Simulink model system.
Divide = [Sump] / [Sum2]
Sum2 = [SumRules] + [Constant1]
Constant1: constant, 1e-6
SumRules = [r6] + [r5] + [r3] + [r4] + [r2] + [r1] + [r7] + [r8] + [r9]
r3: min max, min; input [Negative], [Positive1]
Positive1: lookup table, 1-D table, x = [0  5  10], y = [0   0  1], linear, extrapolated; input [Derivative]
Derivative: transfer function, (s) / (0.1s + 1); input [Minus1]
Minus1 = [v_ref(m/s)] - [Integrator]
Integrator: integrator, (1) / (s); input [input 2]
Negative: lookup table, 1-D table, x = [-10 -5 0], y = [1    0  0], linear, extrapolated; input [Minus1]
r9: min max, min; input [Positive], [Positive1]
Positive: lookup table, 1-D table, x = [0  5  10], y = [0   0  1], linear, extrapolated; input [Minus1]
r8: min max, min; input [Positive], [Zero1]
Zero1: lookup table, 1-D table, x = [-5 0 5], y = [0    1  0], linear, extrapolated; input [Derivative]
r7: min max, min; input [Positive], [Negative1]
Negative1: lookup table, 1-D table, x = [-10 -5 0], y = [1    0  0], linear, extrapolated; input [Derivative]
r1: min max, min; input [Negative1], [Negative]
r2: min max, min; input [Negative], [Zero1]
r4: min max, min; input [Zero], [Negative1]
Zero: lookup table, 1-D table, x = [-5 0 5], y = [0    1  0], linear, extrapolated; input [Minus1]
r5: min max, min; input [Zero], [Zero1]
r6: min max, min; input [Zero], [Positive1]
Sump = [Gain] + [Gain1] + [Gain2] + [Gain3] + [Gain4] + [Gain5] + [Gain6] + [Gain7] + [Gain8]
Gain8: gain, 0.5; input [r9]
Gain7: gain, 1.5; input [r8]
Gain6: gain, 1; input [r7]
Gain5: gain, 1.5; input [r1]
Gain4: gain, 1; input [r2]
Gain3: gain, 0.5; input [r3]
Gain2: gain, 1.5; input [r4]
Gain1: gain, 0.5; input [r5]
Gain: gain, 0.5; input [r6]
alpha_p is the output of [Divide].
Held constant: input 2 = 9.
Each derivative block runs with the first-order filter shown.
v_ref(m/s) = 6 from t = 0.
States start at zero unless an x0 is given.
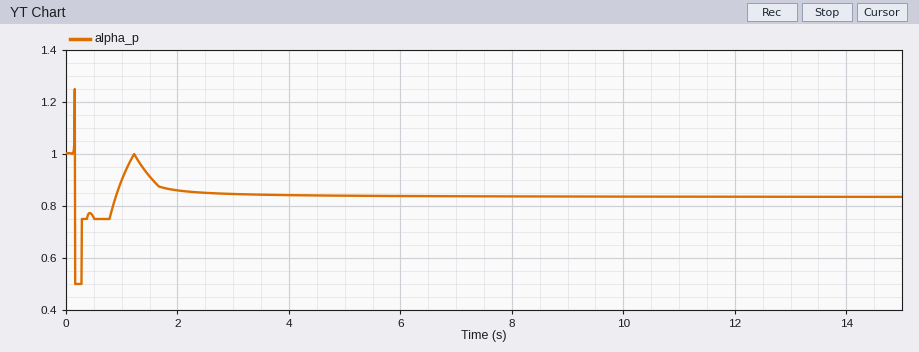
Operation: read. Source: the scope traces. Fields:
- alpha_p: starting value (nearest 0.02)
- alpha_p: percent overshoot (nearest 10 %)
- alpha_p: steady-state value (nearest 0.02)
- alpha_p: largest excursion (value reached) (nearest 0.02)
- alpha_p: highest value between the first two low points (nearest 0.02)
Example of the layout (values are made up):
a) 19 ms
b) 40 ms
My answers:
a) 1.00
b) 200 %
c) 0.84
d) 0.50
e) 0.78
